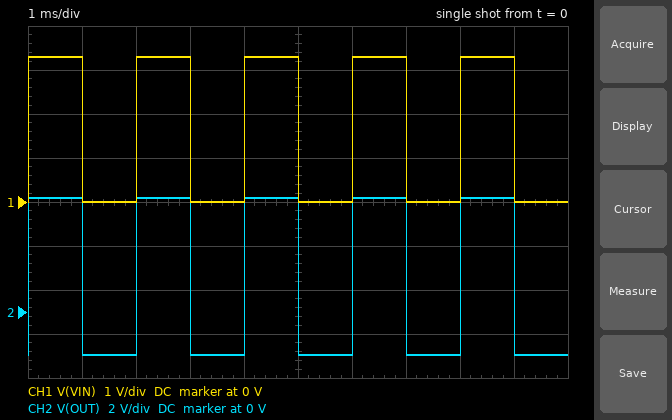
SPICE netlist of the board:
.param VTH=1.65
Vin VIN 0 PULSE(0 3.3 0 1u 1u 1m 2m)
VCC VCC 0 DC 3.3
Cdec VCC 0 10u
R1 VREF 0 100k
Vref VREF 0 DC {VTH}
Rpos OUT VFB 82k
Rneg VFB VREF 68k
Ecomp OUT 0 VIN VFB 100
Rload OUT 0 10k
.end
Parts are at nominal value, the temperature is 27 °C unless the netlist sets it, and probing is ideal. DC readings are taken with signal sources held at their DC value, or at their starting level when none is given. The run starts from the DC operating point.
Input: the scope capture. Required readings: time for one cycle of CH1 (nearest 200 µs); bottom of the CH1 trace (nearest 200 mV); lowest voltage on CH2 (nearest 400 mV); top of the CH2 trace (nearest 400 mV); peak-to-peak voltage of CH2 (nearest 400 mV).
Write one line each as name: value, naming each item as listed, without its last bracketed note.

time for one cycle of CH1: 2.0 ms
bottom of the CH1 trace: 0 V
lowest voltage on CH2: -2.0 V
top of the CH2 trace: 5.2 V
peak-to-peak voltage of CH2: 7.2 V
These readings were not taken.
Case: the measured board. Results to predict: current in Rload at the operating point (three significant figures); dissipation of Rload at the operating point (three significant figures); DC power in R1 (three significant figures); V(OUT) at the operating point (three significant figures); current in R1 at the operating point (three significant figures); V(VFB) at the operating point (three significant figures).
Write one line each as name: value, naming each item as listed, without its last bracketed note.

current in Rload at the operating point: 195 µA
dissipation of Rload at the operating point: 379 µW
DC power in R1: 27.2 µW
V(OUT) at the operating point: -1.95 V
current in R1 at the operating point: 16.5 µA
V(VFB) at the operating point: 19.5 mV
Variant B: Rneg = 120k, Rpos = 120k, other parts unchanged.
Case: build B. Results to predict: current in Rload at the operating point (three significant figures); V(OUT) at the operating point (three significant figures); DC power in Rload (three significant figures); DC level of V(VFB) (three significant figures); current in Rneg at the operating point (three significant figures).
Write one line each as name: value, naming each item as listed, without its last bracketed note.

current in Rload at the operating point: 162 µA
V(OUT) at the operating point: -1.62 V
DC power in Rload: 262 µW
DC level of V(VFB): 16.2 mV
current in Rneg at the operating point: 13.6 µA
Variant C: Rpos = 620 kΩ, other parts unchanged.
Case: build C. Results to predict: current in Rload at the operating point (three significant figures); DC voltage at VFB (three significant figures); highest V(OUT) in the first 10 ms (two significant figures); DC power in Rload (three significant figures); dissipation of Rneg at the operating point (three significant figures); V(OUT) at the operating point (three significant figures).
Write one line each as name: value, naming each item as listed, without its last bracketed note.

current in Rload at the operating point: 1.37 mA
DC voltage at VFB: 137 mV
highest V(OUT) in the first 10 ms: 17 V
DC power in Rload: 18.7 mW
dissipation of Rneg at the operating point: 33.7 µW
V(OUT) at the operating point: -13.7 V
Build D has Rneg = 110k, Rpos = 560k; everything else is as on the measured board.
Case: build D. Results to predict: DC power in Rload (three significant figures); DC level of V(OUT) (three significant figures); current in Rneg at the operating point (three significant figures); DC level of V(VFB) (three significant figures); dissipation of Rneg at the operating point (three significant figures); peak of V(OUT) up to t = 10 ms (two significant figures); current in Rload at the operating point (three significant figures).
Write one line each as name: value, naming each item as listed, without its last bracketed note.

DC power in Rload: 6.27 mW
DC level of V(OUT): -7.92 V
current in Rneg at the operating point: 14.3 µA
DC level of V(VFB): 79.2 mV
dissipation of Rneg at the operating point: 22.4 µW
peak of V(OUT) up to t = 10 ms: 11 V
current in Rload at the operating point: 792 µA
